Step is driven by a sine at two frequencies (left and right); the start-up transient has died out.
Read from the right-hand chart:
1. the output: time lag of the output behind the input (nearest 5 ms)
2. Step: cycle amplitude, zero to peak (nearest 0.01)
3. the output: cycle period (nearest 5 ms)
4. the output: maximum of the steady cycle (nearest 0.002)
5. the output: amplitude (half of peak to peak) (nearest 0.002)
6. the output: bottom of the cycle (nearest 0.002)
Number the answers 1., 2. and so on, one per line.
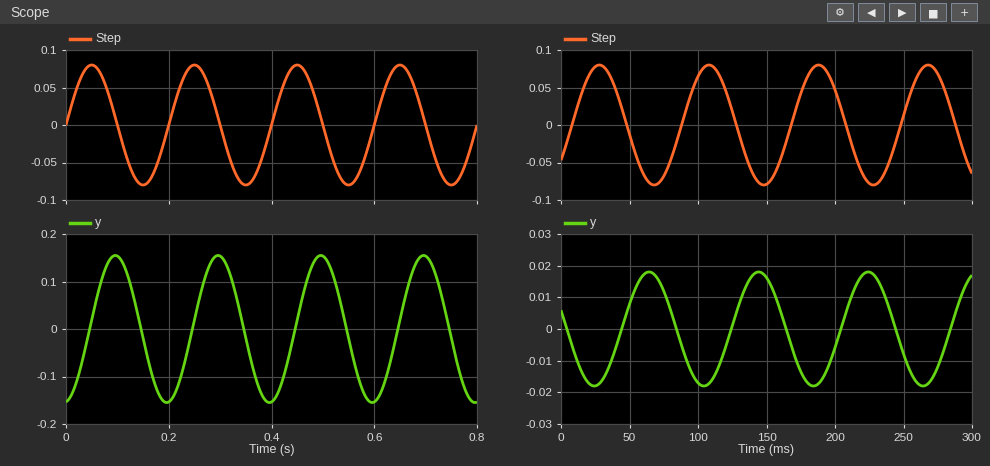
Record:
1. 35 ms
2. 0.08
3. 80 ms
4. 0.018
5. 0.018
6. -0.018
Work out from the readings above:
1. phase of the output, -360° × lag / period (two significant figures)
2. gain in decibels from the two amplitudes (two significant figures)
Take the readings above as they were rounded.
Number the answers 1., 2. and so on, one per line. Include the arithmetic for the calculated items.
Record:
1. -360 × 35 / 80 = -160°
2. 20 log10(0.018 / 0.08) = -13 dB
